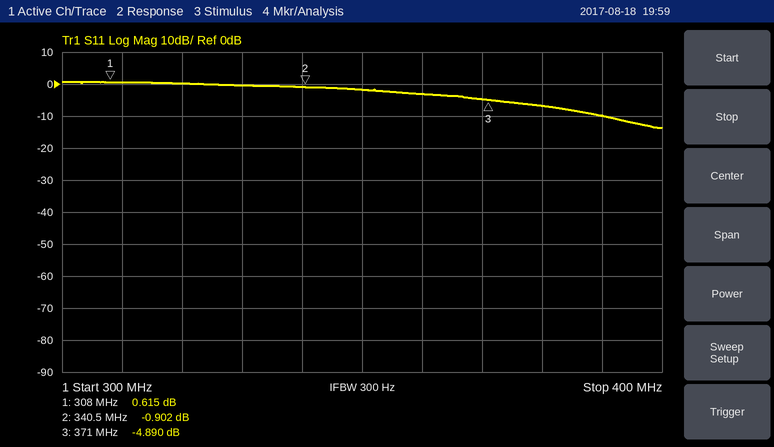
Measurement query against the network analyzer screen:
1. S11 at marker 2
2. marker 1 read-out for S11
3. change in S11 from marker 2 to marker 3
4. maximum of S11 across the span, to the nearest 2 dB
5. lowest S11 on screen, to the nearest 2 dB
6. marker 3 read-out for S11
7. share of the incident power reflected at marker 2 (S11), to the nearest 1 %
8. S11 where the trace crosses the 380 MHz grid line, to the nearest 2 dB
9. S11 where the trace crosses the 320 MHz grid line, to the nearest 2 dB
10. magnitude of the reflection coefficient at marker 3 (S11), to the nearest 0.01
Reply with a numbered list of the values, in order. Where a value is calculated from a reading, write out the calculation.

1. -0.902 dB
2. 0.615 dB
3. -4.89 − (-0.902) = -3.988 dB
4. 0 dB
5. -14 dB
6. -4.890 dB
7. 10^(-0.902/10) ≈ 81 %
8. -6 dB
9. 0 dB
10. 10^(-4.89/20) ≈ 0.57
